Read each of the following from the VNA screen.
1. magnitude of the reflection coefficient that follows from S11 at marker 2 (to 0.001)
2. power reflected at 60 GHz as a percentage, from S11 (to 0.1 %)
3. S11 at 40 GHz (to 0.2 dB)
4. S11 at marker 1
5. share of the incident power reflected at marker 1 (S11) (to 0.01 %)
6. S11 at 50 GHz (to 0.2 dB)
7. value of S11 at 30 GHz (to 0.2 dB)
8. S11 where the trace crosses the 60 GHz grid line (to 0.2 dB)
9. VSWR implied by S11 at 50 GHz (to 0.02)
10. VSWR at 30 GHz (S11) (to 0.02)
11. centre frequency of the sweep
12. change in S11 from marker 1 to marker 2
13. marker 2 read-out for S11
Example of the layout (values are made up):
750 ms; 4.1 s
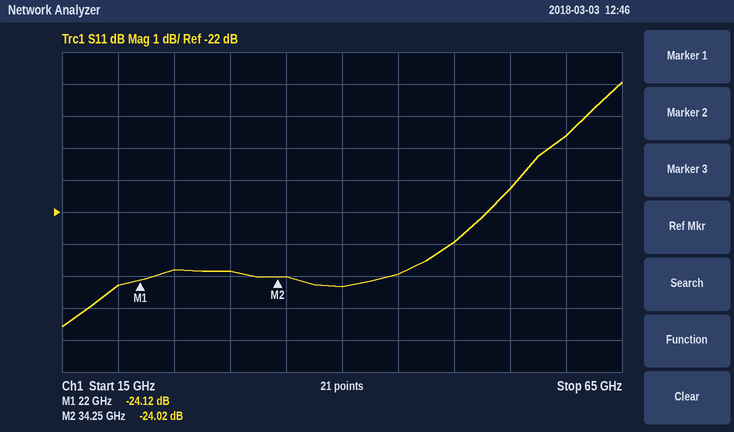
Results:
0.063; 1.1 %; -24.4 dB; -24.12 dB; 0.39 %; -23.0 dB; -23.8 dB; -19.6 dB; 1.16; 1.14; 40 GHz; 0.10 dB; -24.02 dB
